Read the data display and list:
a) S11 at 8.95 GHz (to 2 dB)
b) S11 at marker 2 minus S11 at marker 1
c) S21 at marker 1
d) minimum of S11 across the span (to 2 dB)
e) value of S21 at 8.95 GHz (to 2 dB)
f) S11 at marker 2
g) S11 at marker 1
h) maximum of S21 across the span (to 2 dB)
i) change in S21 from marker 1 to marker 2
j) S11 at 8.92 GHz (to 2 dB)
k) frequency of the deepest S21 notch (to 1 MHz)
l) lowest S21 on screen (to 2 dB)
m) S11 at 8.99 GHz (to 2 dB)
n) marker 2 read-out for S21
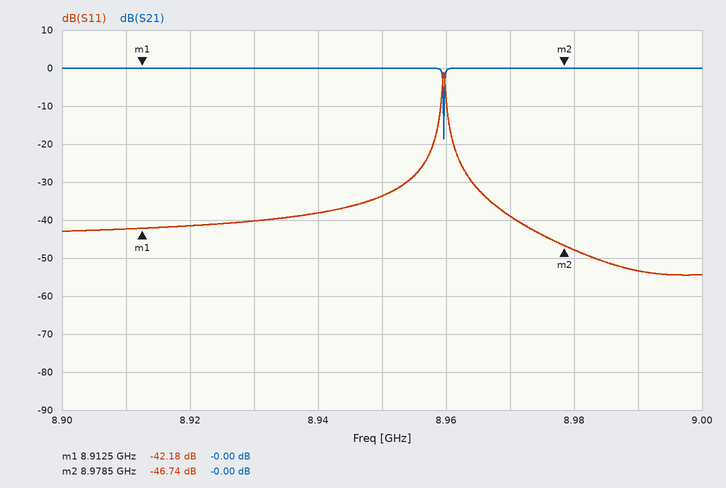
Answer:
-34 dB
-4.56 dB
-0.00 dB
-54 dB
0 dB
-46.74 dB
-42.18 dB
0 dB
0.00 dB
-42 dB
8.960 GHz
-18 dB
-54 dB
-0.00 dB
